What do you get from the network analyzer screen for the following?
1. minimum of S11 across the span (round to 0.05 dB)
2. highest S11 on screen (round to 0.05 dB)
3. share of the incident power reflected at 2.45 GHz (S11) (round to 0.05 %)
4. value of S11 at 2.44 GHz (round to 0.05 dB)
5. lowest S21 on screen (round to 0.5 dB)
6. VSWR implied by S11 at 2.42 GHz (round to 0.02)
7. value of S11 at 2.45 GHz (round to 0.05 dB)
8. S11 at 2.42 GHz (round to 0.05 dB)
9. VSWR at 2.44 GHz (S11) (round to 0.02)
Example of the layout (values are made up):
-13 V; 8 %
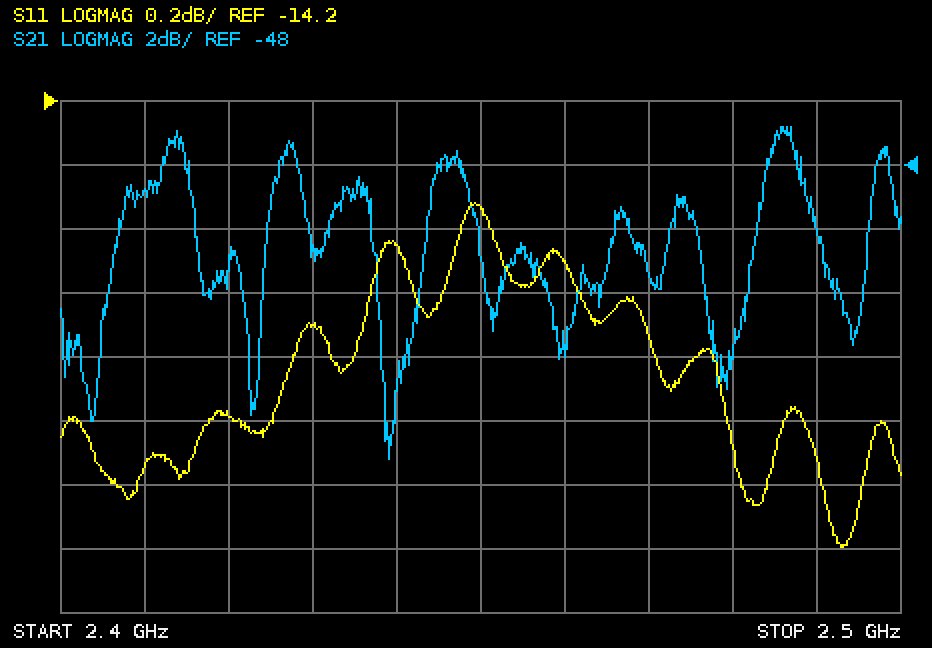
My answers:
-15.60 dB; -14.50 dB; 3.50 %; -14.65 dB; -57.0 dB; 1.42; -14.55 dB; -15.20 dB; 1.46
